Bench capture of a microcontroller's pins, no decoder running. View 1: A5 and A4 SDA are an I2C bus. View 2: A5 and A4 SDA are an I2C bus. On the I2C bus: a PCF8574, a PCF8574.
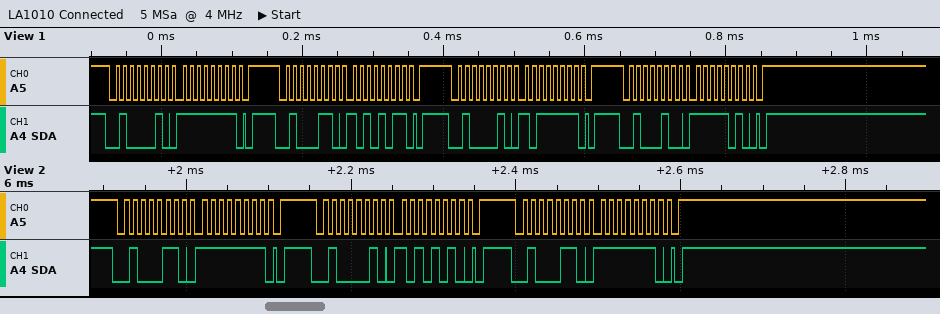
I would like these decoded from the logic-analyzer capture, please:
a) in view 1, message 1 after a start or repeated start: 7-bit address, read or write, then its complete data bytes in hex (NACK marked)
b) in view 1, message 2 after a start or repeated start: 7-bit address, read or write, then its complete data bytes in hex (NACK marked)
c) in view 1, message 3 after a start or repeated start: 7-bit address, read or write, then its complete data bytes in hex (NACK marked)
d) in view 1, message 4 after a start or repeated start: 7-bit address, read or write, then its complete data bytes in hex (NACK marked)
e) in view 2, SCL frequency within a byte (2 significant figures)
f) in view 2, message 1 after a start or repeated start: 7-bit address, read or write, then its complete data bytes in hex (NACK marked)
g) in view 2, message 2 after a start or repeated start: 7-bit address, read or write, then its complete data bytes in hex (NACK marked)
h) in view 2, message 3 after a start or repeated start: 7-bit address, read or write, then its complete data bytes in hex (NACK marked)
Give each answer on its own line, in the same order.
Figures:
0x21 write: FF
0x23 write: AB
0x21 write: BF
0x22 write: FA
100 kHz
0x23 write: FF
0x21 write: AA
0x23 write: FE
